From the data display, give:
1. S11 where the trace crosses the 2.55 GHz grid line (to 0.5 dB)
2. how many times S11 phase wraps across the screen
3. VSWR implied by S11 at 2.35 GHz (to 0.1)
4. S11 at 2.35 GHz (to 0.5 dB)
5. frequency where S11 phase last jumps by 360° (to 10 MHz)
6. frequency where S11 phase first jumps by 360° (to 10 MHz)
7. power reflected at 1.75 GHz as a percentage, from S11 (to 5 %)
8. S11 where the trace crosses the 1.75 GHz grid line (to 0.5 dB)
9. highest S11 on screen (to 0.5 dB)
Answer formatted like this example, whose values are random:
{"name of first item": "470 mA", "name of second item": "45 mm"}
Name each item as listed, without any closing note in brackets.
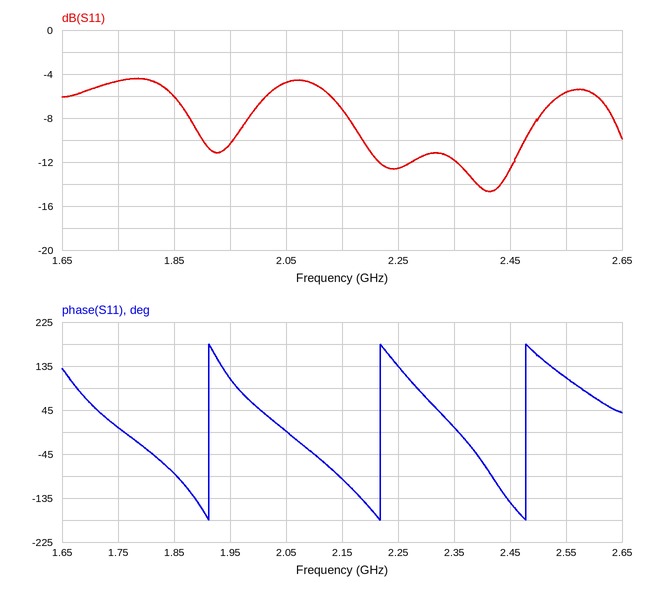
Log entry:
{"S11 where the trace crosses the 2.55 GHz grid line": "-5.5 dB", "how many times S11 phase wraps across the screen": "3", "VSWR implied by S11 at 2.35 GHz": "1.7", "S11 at 2.35 GHz": "-12.0 dB", "frequency where S11 phase last jumps by 360°": "2.48 GHz", "frequency where S11 phase first jumps by 360°": "1.91 GHz", "power reflected at 1.75 GHz as a percentage, from S11": "35 %", "S11 where the trace crosses the 1.75 GHz grid line": "-4.5 dB", "highest S11 on screen": "-4.5 dB"}
